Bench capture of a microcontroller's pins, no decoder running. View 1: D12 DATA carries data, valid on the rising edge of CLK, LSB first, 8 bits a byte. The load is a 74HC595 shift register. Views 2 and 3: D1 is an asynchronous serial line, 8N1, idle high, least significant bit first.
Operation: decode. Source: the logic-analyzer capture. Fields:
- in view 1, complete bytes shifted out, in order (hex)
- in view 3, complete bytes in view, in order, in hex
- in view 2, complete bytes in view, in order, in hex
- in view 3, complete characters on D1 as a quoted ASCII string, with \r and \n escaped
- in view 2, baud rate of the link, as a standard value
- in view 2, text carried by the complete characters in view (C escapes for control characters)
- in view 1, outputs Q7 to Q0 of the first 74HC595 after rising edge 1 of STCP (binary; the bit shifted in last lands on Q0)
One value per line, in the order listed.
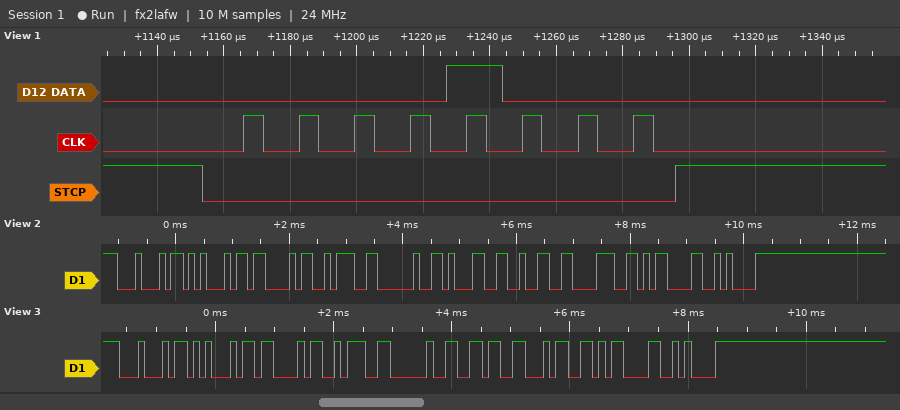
10
44 45 43 3A 20 36 34 0D 0A
44 45 43 3A 20 31 32 38 0D 0A
"DEC: 64\r\n"
9600 baud
"DEC: 128\r\n"
00001000
